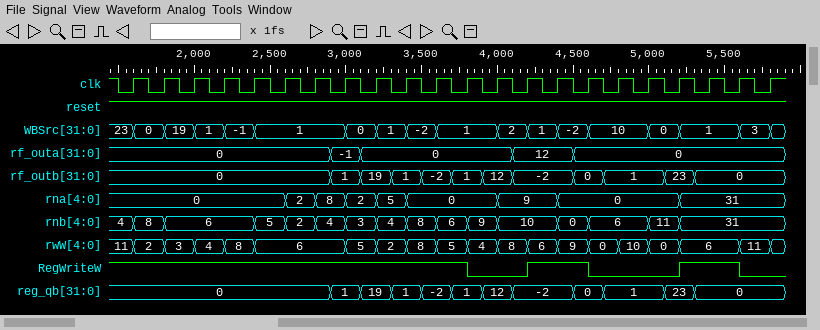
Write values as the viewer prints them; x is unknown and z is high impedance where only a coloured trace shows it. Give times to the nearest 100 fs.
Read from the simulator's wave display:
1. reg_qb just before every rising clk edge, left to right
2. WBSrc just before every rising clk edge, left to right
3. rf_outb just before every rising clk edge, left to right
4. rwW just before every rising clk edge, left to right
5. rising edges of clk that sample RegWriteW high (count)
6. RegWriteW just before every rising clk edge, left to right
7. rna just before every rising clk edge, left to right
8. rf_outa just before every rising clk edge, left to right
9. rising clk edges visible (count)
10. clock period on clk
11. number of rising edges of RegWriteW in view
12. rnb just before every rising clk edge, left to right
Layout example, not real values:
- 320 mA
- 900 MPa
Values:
- 0, 0, 0, 0, 0, 0, 0, 1, 19, 1, -2, 1, 12, -2, -2, 0, 1, 1, 23, 0, 0, 0
- 23, 0, 19, 1, -1, 1, 1, 1, 0, 1, -2, 1, 1, 2, 1, -2, 10, 10, 0, 1, 1, 3
- 0, 0, 0, 0, 0, 0, 0, 1, 19, 1, -2, 1, 12, -2, -2, 0, 1, 1, 23, 0, 0, 0
- 11, 2, 3, 4, 8, 6, 6, 6, 5, 2, 8, 5, 4, 8, 6, 9, 0, 10, 0, 6, 6, 11
- 16
- 1 1 1 1 1 1 1 1 1 1 1 1 0 0 1 1 0 0 0 1 1 0
- 0, 0, 0, 0, 0, 0, 2, 8, 2, 5, 0, 0, 0, 9, 9, 0, 0, 0, 0, 31, 31, 31
- 0, 0, 0, 0, 0, 0, 0, -1, 0, 0, 0, 0, 0, 12, 12, 0, 0, 0, 0, 0, 0, 0
- 22
- 200 fs
- 2
- 4, 8, 6, 6, 6, 5, 2, 4, 3, 4, 8, 6, 9, 10, 10, 0, 6, 6, 11, 31, 31, 31
